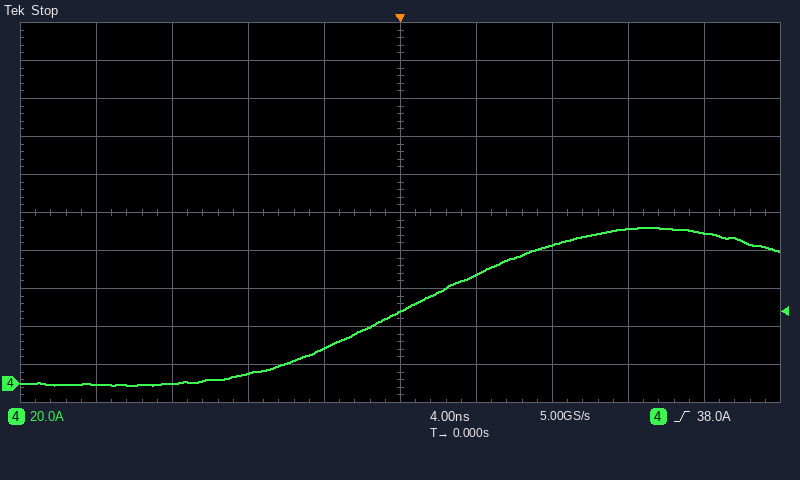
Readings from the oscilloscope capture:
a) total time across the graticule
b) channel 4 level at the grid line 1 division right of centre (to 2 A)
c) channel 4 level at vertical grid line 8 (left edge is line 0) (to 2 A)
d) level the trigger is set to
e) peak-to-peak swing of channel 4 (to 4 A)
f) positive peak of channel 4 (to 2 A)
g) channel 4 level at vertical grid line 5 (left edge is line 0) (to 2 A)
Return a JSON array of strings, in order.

["40 ns", "58 A", "82 A", "38.0 A", "84 A", "82 A", "38 A"]
